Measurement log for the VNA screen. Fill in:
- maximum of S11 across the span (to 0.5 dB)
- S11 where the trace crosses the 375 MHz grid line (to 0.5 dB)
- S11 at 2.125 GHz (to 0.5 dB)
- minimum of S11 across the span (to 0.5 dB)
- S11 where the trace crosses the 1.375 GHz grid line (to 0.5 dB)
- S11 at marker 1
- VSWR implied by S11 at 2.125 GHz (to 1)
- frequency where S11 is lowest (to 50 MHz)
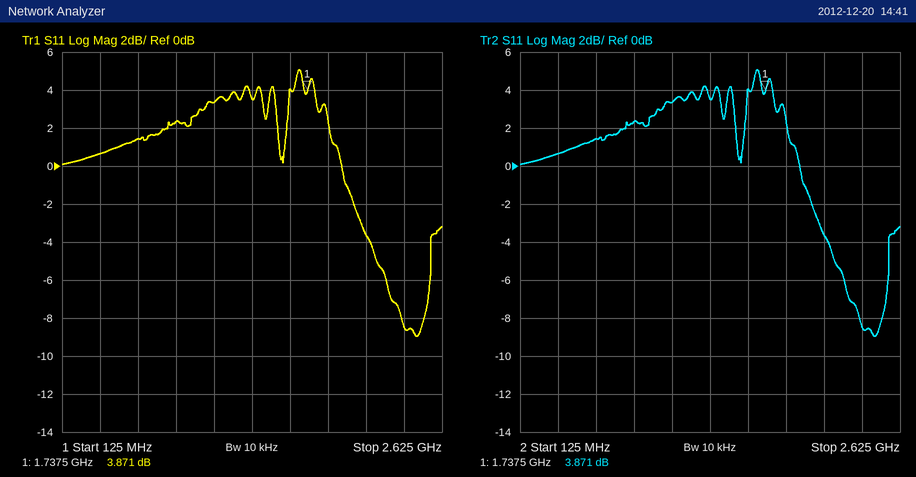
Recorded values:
5.0 dB
0.5 dB
-3.5 dB
-9.0 dB
3.5 dB
3.871 dB
5
2.45 GHz
